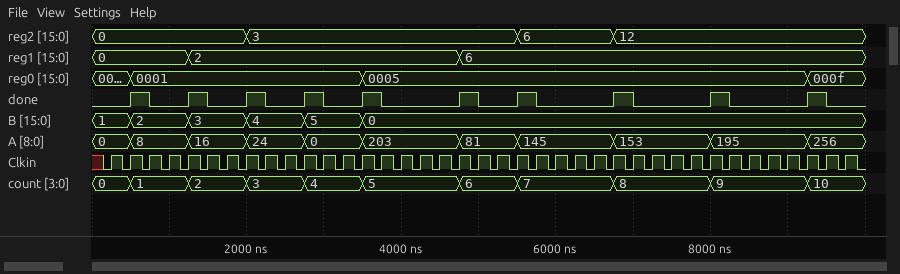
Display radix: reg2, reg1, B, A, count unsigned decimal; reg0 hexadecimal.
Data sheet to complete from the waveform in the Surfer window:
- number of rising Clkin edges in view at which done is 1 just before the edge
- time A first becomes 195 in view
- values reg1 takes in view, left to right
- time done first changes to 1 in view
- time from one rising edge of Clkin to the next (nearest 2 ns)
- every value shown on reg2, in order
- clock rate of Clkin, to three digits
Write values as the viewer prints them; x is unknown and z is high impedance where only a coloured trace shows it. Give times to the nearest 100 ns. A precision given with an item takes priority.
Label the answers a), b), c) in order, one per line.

a) 10
b) 8000 ns
c) 0, 2, 6
d) 500 ns
e) 250 ns
f) 0, 3, 6, 12
g) 4.00 MHz
